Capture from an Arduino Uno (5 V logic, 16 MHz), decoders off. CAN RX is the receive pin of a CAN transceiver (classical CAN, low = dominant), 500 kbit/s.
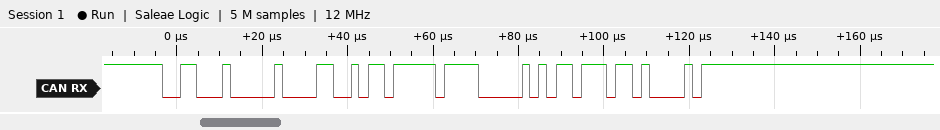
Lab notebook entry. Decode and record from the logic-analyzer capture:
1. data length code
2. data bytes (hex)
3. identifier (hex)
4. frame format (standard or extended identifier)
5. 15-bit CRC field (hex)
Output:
3
2D FF 02
0x310
standard
0x6ED0
